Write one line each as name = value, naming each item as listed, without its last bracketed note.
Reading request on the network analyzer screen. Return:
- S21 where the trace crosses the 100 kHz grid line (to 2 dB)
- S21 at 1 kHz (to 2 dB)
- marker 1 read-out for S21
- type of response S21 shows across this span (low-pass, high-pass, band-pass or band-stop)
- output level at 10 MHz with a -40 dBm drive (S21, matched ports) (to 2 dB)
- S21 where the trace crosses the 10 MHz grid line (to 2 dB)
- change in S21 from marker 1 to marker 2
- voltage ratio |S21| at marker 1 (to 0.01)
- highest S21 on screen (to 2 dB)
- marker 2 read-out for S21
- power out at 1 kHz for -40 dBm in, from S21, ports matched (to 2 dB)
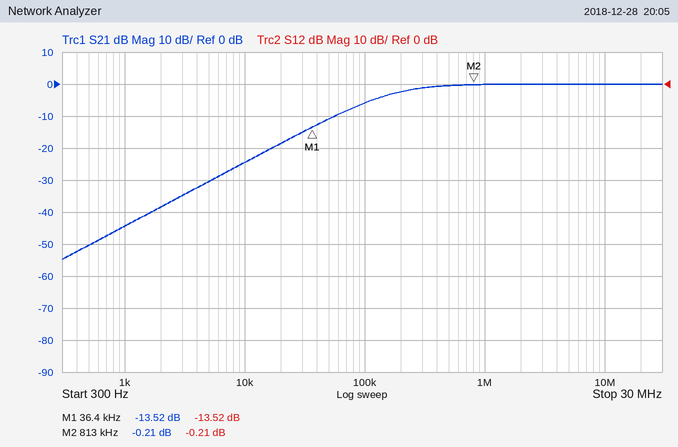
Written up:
S21 where the trace crosses the 100 kHz grid line = -6 dB
S21 at 1 kHz = -44 dB
marker 1 read-out for S21 = -13.52 dB
type of response S21 shows across this span = high-pass
output level at 10 MHz with a -40 dBm drive (S21, matched ports) = -40 dBm
S21 where the trace crosses the 10 MHz grid line = 0 dB
change in S21 from marker 1 to marker 2 = 13.31 dB
voltage ratio |S21| at marker 1 = 0.21
highest S21 on screen = 0 dB
marker 2 read-out for S21 = -0.21 dB
power out at 1 kHz for -40 dBm in, from S21, ports matched = -84 dBm
